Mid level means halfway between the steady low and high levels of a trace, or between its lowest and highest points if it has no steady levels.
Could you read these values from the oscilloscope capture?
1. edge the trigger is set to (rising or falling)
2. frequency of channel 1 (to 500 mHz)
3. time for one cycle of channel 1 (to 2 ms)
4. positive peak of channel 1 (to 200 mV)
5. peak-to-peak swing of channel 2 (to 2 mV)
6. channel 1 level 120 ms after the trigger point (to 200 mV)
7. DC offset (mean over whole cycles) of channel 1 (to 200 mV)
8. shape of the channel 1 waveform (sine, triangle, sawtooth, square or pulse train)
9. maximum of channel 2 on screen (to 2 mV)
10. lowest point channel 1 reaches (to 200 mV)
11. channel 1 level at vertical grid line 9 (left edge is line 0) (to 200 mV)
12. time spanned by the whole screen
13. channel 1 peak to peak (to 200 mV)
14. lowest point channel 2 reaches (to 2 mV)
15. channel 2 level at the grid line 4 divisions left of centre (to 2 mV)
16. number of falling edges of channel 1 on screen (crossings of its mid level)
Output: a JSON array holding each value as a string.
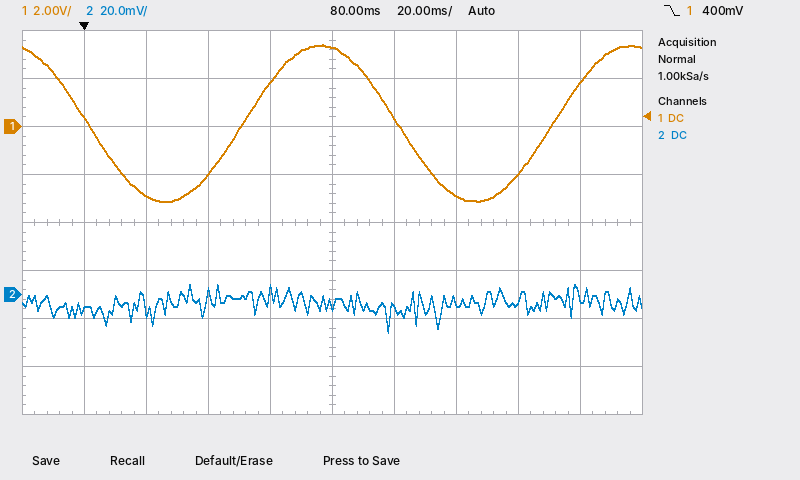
["falling", "10.0 Hz", "100 ms", "3.4 V", "20 mV", "-2.8 V", "200 mV", "sine", "4 mV", "-3.2 V", "1.8 V", "200 ms", "6.6 V", "-16 mV", "-6 mV", "2"]
